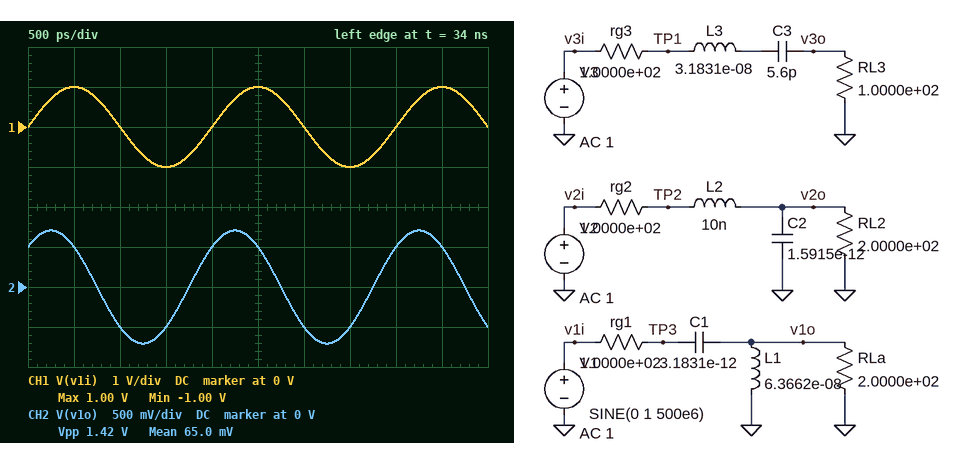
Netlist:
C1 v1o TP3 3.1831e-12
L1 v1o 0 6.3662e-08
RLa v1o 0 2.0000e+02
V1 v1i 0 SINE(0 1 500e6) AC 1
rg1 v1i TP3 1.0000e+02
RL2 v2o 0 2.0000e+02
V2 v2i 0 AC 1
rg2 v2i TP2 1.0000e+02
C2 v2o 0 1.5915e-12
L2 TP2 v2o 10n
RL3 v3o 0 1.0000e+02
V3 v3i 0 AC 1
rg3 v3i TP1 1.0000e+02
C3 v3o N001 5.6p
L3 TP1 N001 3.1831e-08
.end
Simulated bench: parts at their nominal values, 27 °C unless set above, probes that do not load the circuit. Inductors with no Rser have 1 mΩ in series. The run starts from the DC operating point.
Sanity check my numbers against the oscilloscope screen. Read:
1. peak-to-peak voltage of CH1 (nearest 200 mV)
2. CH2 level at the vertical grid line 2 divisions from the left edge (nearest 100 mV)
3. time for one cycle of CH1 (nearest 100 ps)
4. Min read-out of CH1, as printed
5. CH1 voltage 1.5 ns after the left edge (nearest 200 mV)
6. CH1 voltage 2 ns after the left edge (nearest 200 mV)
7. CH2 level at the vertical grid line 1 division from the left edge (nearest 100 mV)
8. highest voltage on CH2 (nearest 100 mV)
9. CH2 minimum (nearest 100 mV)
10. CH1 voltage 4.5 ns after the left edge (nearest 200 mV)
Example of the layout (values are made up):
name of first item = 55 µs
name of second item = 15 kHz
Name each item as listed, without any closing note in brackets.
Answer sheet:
peak-to-peak voltage of CH1 = 2.0 V
CH2 level at the vertical grid line 2 divisions from the left edge = -500 mV
time for one cycle of CH1 = 2.0 ns
Min read-out of CH1, as printed = -1.00 V
CH1 voltage 1.5 ns after the left edge = -1.0 V
CH1 voltage 2 ns after the left edge = 0 V
CH2 level at the vertical grid line 1 division from the left edge = 500 mV
highest voltage on CH2 = 700 mV
CH2 minimum = -700 mV
CH1 voltage 4.5 ns after the left edge = 1.0 V
